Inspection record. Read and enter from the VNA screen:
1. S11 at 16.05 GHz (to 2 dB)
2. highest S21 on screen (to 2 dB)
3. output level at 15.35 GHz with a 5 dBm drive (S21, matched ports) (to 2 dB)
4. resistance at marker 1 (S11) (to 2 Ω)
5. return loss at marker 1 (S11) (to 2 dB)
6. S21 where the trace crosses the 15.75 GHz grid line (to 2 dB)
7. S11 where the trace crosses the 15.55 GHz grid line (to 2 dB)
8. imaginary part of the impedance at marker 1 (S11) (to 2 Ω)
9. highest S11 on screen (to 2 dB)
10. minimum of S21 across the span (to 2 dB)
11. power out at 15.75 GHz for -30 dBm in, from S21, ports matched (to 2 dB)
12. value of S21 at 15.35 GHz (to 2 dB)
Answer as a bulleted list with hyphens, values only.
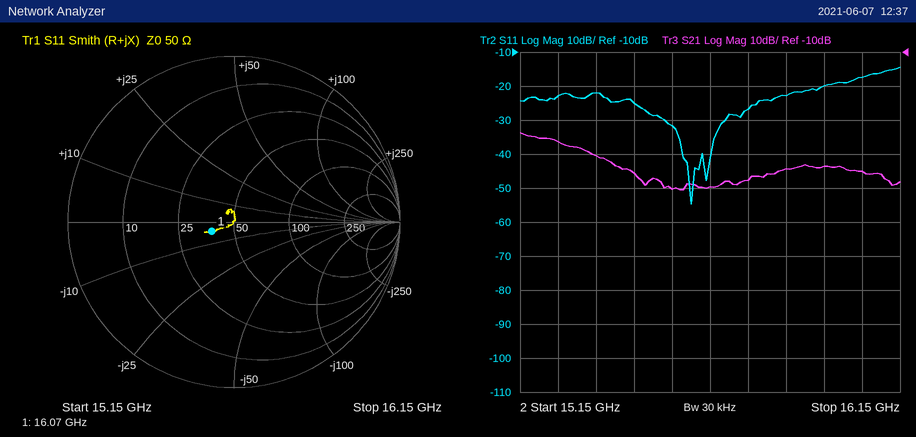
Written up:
- -18 dB
- -34 dB
- -36 dBm
- 38 Ω
- 16 dB
- -48 dB
- -32 dB
- -4 Ω
- -14 dB
- -50 dB
- -78 dBm
- -40 dB
